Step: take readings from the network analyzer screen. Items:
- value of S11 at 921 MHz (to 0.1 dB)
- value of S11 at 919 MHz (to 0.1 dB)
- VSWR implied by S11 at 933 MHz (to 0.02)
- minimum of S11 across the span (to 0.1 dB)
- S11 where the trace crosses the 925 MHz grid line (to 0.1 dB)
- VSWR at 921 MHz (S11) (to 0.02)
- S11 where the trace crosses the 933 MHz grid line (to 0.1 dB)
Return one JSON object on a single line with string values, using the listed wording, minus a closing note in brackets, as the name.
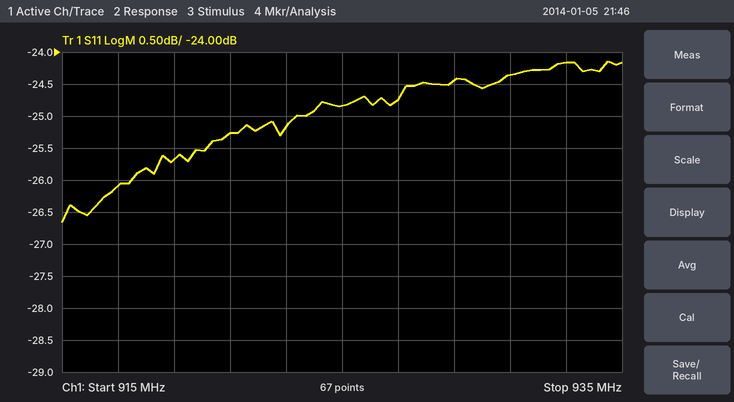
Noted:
{"value of S11 at 921 MHz": "-25.3 dB", "value of S11 at 919 MHz": "-25.7 dB", "VSWR implied by S11 at 933 MHz": "1.14", "minimum of S11 across the span": "-26.7 dB", "S11 where the trace crosses the 925 MHz grid line": "-24.8 dB", "VSWR at 921 MHz (S11)": "1.12", "S11 where the trace crosses the 933 MHz grid line": "-24.2 dB"}
